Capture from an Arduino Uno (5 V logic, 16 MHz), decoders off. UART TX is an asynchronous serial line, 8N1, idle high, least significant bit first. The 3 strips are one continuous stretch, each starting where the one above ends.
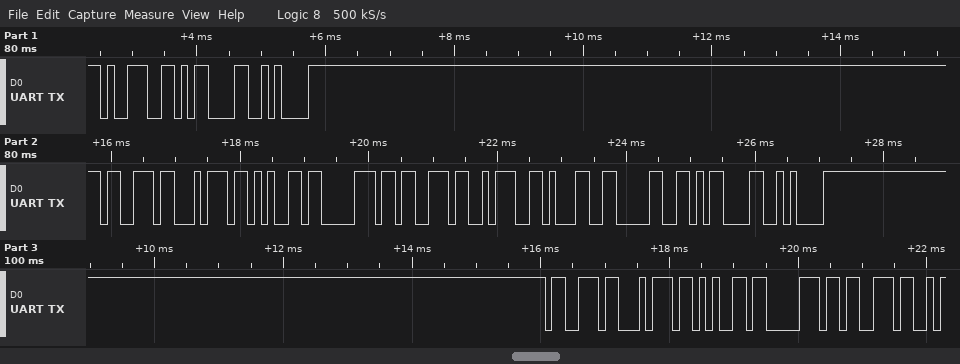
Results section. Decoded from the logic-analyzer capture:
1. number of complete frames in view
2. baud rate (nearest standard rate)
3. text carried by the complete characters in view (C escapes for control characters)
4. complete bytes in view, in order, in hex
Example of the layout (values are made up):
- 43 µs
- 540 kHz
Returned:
- 18
- 9600 baud
- "9\r\nsteps:10\r\nsteps"
- 39 0D 0A 73 74 65 70 73 3A 31 30 0D 0A 73 74 65 70 73
